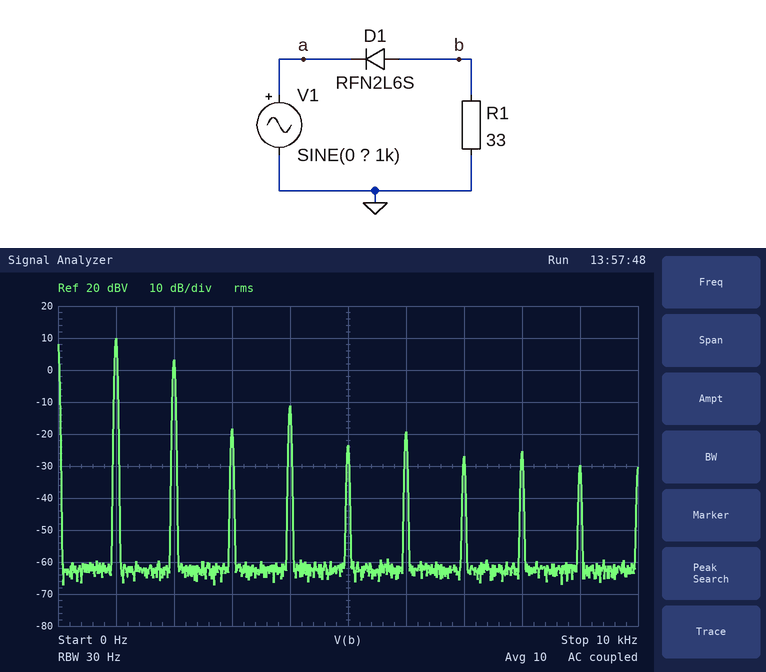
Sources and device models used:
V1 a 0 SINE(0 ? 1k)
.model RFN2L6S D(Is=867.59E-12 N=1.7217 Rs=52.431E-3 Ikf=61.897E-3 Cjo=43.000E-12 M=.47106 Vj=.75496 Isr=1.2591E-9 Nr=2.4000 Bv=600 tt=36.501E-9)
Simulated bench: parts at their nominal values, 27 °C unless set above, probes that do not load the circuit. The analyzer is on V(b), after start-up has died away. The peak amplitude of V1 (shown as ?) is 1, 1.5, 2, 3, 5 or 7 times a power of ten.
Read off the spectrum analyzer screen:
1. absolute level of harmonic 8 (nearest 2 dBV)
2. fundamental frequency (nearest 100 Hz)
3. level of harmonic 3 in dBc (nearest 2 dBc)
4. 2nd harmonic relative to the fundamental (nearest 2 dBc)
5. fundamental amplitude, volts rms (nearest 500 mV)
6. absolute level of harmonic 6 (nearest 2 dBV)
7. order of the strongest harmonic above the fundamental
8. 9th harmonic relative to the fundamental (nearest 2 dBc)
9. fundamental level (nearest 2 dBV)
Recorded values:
-26 dBV
1.0 kHz
-28 dBc
-6 dBc
3.0 V
-20 dBV
2
-40 dBc
10 dBV
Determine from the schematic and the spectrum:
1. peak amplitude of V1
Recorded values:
10 V
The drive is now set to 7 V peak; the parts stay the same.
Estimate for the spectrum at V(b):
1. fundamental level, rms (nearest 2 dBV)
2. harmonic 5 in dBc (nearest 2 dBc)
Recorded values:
6 dBV
-30 dBc
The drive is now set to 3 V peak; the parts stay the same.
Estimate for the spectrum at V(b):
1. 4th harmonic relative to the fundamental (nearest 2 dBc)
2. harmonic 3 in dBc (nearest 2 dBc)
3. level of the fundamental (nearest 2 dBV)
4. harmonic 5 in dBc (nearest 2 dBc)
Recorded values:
-24 dBc
-18 dBc
-4 dBV
-24 dBc
